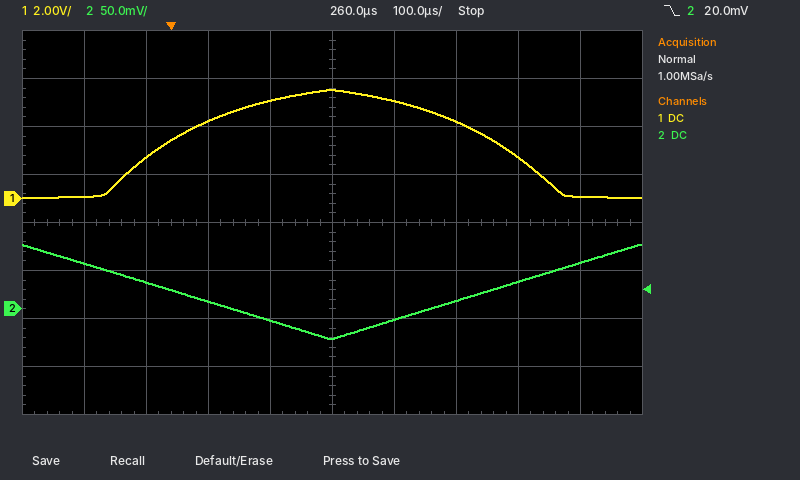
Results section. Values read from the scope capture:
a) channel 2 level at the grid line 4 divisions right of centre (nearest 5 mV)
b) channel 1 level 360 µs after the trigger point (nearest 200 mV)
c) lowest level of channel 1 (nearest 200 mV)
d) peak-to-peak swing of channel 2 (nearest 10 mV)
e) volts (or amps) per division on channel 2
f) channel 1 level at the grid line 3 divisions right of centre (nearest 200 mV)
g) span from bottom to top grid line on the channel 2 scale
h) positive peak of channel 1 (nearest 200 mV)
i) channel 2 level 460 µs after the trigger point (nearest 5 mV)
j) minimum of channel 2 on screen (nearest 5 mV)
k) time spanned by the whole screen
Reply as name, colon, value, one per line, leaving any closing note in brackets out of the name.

channel 2 level at the grid line 4 divisions right of centre: 50 mV
channel 1 level 360 µs after the trigger point: 4.0 V
lowest level of channel 1: 0.0 V
peak-to-peak swing of channel 2: 100 mV
volts (or amps) per division on channel 2: 50 mV
channel 1 level at the grid line 3 divisions right of centre: 1.8 V
span from bottom to top grid line on the channel 2 scale: 400 mV
positive peak of channel 1: 4.6 V
channel 2 level 460 µs after the trigger point: 10 mV
minimum of channel 2 on screen: -30 mV
time spanned by the whole screen: 1 ms
